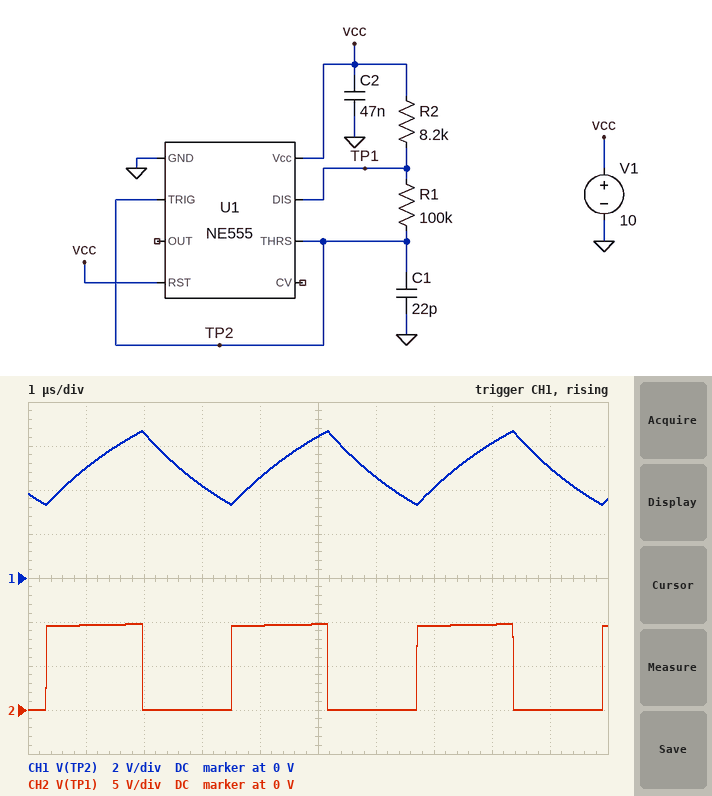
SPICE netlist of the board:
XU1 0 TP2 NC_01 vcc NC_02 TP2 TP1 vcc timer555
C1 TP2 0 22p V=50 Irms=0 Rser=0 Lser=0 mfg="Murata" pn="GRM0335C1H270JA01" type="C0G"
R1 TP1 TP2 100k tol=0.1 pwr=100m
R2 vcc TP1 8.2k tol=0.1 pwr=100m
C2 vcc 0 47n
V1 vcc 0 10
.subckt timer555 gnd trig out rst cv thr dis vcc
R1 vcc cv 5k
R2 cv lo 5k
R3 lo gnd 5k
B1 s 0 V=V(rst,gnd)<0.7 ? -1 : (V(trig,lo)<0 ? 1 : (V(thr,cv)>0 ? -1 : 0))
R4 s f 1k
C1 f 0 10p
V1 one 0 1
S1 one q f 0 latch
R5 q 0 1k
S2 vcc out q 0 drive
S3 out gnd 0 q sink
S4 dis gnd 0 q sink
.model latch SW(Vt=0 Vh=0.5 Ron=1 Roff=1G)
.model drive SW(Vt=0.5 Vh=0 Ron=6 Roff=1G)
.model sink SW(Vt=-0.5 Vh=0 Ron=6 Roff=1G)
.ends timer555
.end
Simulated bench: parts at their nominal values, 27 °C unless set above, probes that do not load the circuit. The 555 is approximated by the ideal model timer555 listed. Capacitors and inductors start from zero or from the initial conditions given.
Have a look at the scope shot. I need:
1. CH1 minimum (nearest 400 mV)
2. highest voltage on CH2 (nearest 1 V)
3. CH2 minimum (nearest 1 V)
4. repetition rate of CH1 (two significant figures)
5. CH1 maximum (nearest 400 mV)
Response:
3.2 V
10 V
0 V
310 kHz
6.8 V
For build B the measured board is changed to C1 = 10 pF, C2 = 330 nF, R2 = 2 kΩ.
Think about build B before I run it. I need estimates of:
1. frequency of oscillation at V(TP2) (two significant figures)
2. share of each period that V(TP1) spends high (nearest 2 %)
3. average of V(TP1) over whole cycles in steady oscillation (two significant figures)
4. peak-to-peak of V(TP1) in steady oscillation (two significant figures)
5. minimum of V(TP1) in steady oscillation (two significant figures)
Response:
700 kHz
50 %
5.0 V
9.9 V
30 mV
